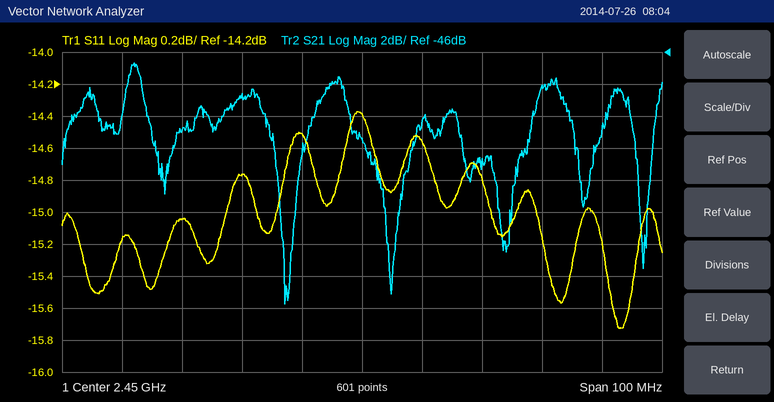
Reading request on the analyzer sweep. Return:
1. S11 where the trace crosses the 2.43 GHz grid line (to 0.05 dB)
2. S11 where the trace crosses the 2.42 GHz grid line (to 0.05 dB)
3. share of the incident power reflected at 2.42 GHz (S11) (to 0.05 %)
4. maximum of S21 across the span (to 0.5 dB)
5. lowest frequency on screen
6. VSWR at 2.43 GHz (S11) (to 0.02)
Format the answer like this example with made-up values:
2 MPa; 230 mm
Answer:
-14.75 dB; -15.05 dB; 3.15 %; -46.5 dB; 2.4 GHz; 1.44
